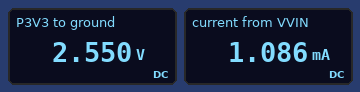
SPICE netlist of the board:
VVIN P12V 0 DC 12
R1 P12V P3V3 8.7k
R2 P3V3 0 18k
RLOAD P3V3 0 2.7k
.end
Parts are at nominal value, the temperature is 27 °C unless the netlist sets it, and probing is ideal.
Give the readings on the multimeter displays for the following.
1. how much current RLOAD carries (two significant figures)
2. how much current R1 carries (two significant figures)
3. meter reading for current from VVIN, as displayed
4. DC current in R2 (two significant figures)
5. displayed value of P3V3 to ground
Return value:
940 µA
1.1 mA
1.086 mA
140 µA
2.550 V
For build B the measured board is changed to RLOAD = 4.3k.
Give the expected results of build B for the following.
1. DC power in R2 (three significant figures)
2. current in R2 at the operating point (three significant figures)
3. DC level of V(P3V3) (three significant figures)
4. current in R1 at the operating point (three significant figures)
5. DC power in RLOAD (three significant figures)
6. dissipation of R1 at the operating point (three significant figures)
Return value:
651 µW
190 µA
3.42 V
986 µA
2.72 mW
8.46 mW
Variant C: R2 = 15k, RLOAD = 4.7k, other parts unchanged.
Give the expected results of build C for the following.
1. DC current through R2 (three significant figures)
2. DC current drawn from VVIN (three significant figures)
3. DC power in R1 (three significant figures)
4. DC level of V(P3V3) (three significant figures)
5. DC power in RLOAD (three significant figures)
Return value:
233 µA
977 µA
8.31 mW
3.50 V
2.60 mW
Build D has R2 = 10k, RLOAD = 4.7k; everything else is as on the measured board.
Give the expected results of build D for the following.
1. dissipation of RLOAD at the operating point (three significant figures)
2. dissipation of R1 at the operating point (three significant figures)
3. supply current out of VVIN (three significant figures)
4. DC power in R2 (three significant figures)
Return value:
2.21 mW
8.85 mW
1.01 mA
1.04 mW
